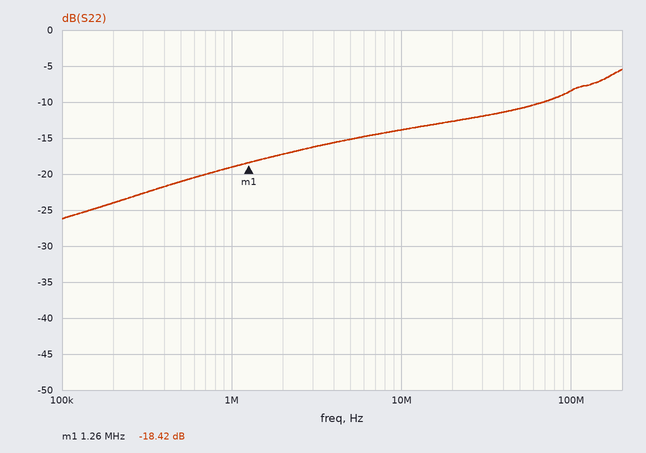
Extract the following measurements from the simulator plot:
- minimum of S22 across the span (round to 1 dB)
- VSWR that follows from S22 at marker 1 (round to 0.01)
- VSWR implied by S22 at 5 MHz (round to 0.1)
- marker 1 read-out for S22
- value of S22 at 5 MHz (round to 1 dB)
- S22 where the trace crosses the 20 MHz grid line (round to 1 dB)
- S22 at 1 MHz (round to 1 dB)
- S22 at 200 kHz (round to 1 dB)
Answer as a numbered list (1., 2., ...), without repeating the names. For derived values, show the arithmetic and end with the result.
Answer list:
1. -26 dB
2. (1 + 0.1199)/(1 − 0.1199) ≈ 1.27
3. |Γ| = 10^(-15/20) = 0.1778; VSWR = (1 + 0.1778)/(1 − 0.1778) ≈ 1.4
4. -18.42 dB
5. -15 dB
6. -13 dB
7. -19 dB
8. -24 dB
